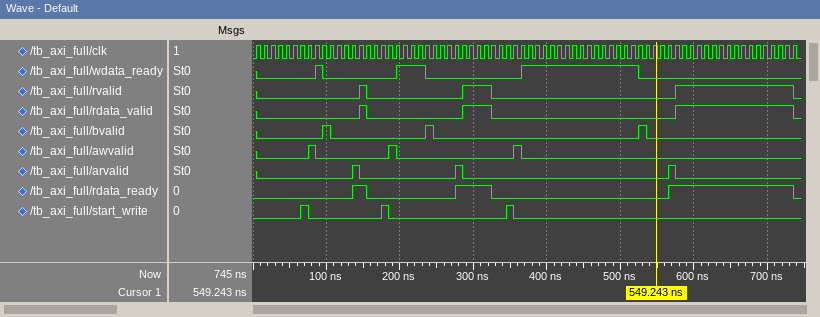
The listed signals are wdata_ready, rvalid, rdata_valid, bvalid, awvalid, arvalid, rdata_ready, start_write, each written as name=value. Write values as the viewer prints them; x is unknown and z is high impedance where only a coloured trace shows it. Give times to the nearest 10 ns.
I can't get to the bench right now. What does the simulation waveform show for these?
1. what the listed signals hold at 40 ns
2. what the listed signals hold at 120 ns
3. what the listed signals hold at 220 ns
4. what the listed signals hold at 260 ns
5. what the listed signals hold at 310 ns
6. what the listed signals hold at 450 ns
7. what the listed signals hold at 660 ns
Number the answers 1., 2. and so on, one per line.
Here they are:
1. wdata_ready=0, rvalid=0, rdata_valid=0, bvalid=0, awvalid=0, arvalid=0, rdata_ready=0, start_write=0
2. wdata_ready=0, rvalid=0, rdata_valid=0, bvalid=0, awvalid=0, arvalid=0, rdata_ready=0, start_write=0
3. wdata_ready=1, rvalid=0, rdata_valid=0, bvalid=0, awvalid=0, arvalid=0, rdata_ready=0, start_write=0
4. wdata_ready=0, rvalid=0, rdata_valid=0, bvalid=0, awvalid=0, arvalid=0, rdata_ready=0, start_write=0
5. wdata_ready=0, rvalid=1, rdata_valid=1, bvalid=0, awvalid=0, arvalid=0, rdata_ready=1, start_write=0
6. wdata_ready=1, rvalid=0, rdata_valid=0, bvalid=0, awvalid=0, arvalid=0, rdata_ready=0, start_write=0
7. wdata_ready=0, rvalid=1, rdata_valid=1, bvalid=0, awvalid=0, arvalid=0, rdata_ready=1, start_write=0
